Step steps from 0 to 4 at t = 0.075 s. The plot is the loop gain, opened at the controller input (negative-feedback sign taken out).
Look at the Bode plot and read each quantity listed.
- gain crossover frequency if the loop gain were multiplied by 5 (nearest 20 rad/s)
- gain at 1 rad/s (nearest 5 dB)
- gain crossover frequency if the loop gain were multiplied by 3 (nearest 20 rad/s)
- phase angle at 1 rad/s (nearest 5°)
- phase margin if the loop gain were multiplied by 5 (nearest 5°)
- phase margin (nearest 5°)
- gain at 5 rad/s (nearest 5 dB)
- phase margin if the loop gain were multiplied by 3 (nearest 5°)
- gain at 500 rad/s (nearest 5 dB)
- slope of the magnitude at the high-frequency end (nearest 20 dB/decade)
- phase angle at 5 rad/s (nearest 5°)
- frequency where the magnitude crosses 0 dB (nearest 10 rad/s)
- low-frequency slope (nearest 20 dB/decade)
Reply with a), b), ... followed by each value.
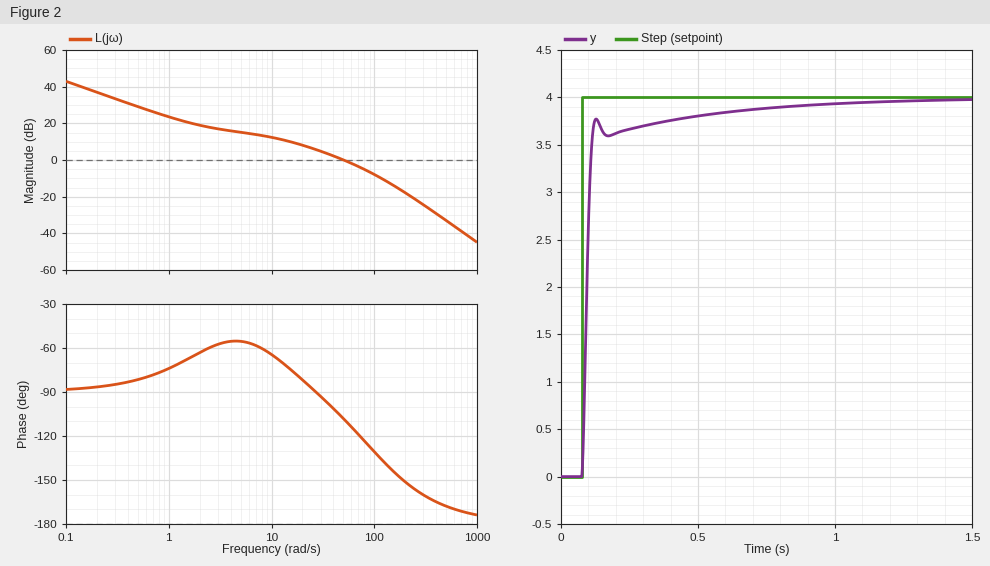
a) 160 rad/s
b) 25 dB
c) 120 rad/s
d) -75°
e) 35°
f) 70°
g) 15 dB
h) 45°
i) -35 dB
j) -40 dB/decade
k) -55°
l) 50 rad/s
m) -20 dB/decade
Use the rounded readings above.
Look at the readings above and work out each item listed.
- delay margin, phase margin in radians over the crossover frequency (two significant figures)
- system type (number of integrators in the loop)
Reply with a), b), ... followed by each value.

a) 0.024 s
b) 1
